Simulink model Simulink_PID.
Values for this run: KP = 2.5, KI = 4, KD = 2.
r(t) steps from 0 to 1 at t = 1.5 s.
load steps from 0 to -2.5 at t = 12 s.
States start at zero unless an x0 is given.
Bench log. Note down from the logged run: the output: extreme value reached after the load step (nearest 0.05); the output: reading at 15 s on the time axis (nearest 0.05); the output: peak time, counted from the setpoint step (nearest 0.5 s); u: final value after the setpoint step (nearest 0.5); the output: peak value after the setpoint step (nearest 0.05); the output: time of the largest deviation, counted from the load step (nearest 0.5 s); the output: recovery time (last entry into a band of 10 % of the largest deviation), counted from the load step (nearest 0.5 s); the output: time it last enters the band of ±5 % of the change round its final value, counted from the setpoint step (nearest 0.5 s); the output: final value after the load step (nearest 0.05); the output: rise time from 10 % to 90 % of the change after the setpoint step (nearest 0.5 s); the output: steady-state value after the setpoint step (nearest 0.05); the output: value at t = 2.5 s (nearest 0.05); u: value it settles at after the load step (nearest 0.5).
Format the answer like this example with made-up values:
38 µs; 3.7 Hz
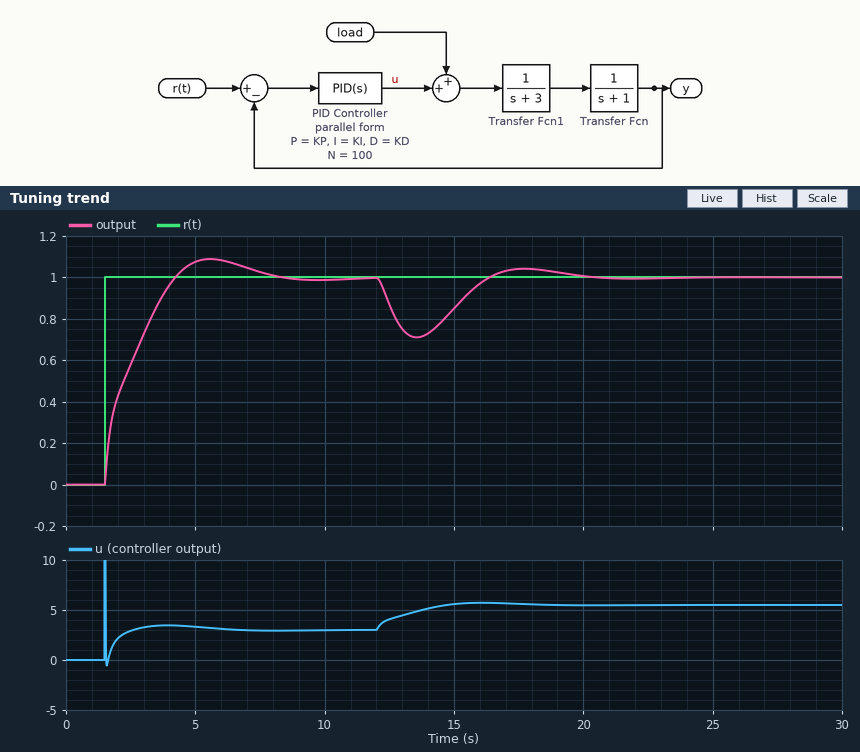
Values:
0.70; 0.85; 4.0 s; 3.0; 1.10; 1.5 s; 7.0 s; 5.5 s; 1.00; 2.0 s; 1.00; 0.60; 5.5
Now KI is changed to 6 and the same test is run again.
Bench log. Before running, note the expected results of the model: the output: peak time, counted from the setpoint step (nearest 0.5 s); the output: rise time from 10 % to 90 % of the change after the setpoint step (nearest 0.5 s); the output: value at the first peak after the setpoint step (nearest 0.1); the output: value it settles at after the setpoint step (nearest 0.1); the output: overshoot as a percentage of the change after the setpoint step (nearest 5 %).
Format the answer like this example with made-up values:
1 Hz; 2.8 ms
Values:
3.0 s; 1.5 s; 1.2; 1.0; 15 %
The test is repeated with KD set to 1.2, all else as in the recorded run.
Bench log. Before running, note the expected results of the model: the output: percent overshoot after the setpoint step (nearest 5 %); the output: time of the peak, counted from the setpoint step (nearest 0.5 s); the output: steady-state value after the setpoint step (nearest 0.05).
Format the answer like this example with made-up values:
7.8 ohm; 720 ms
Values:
10 %; 3.5 s; 1.00
